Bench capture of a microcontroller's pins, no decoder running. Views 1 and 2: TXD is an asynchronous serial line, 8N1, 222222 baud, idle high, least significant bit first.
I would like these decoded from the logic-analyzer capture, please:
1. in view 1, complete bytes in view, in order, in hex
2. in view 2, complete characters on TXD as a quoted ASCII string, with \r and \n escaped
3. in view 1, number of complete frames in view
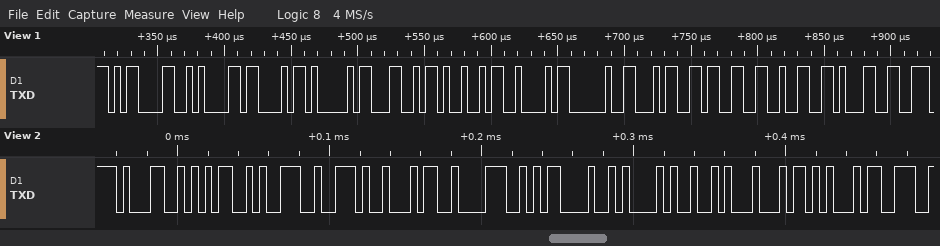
0D 0A 43 41 4C 49 42 20 34 33 32 31
"159.48\r\nIDE"
12
